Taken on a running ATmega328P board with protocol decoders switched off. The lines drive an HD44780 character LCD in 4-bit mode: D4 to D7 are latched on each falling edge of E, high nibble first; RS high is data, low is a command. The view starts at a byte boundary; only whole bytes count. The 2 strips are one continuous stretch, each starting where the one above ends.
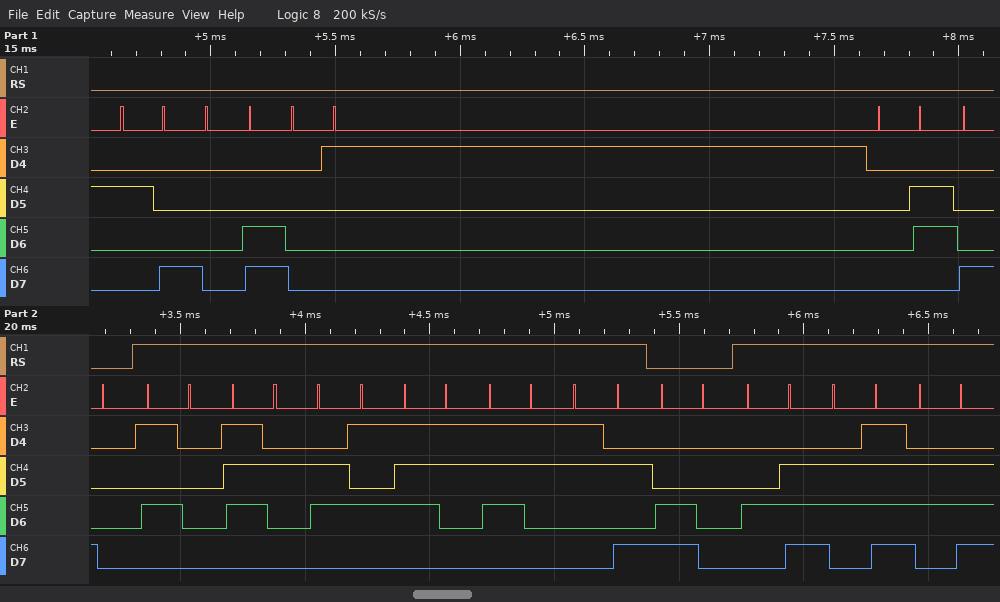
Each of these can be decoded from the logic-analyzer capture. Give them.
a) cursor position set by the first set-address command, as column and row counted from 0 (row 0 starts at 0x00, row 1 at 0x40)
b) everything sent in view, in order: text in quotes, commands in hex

column 0, row 0
0x28 0x0C 0x01 0x06 0x80 "Press:" 0xC0 "Non"
